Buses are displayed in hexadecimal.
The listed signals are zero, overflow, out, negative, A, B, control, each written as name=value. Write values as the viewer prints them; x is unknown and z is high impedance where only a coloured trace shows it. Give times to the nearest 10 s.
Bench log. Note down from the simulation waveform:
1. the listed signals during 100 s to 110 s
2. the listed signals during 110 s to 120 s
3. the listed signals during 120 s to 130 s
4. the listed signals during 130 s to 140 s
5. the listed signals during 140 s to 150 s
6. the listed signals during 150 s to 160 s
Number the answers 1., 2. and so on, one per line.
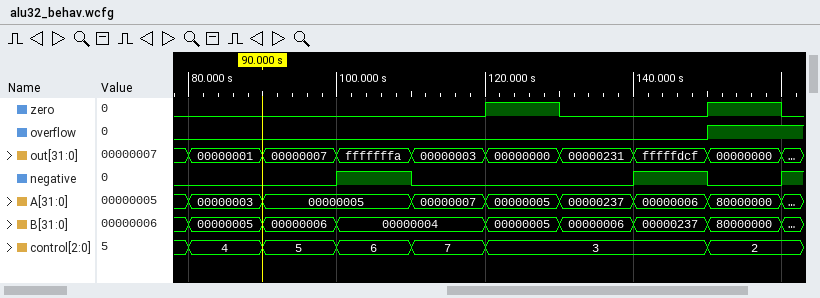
1. zero=0, overflow=0, out=fffffffa, negative=1, A=00000005, B=00000004, control=6
2. zero=0, overflow=0, out=00000003, negative=0, A=00000007, B=00000004, control=7
3. zero=1, overflow=0, out=00000000, negative=0, A=00000005, B=00000005, control=3
4. zero=0, overflow=0, out=00000231, negative=0, A=00000237, B=00000006, control=3
5. zero=0, overflow=0, out=fffffdcf, negative=1, A=00000006, B=00000237, control=3
6. zero=1, overflow=1, out=00000000, negative=0, A=80000000, B=80000000, control=2
